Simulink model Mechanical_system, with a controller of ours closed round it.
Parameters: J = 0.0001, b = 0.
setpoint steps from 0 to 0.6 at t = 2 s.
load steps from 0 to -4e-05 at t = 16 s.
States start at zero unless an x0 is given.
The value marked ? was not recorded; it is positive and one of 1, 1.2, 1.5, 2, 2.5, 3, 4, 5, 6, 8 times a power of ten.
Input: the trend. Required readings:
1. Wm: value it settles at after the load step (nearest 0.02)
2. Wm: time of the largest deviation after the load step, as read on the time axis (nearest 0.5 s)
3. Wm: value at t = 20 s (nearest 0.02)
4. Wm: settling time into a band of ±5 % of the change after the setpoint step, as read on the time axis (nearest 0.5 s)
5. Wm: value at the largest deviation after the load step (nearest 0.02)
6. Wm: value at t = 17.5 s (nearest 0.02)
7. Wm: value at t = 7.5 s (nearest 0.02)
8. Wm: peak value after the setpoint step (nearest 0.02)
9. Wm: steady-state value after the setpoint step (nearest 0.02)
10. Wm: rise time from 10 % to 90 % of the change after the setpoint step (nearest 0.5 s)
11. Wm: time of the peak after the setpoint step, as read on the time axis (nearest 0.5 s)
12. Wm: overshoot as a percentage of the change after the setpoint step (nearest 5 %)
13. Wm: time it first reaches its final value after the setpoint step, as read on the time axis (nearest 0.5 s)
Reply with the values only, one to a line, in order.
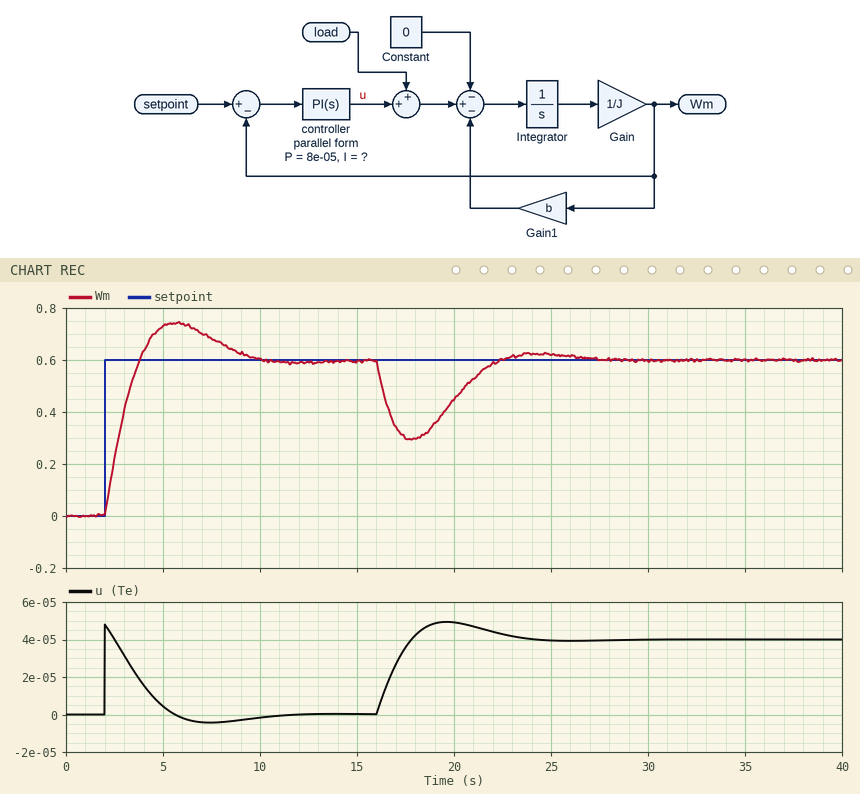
0.60
18.0 s
0.44
9.0 s
0.30
0.30
0.68
0.74
0.60
1.5 s
5.5 s
25 %
4.0 s
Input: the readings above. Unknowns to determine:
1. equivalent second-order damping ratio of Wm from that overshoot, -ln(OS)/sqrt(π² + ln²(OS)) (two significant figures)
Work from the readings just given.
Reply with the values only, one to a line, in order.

0.40
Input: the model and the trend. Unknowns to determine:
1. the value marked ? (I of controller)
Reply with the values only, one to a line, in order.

4e-05
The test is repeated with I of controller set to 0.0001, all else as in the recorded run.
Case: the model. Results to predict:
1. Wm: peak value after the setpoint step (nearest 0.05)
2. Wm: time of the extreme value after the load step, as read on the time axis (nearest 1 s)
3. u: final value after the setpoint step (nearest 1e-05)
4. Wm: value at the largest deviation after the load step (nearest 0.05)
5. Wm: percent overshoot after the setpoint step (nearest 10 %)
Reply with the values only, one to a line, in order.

0.80
17 s
0.00000
0.35
40 %
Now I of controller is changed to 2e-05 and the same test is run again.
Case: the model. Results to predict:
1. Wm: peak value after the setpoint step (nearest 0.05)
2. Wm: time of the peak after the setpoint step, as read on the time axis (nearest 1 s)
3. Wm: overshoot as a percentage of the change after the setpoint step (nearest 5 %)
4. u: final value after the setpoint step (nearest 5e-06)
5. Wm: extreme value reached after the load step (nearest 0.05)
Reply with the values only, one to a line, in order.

0.70
7 s
15 %
0.000000
0.25
